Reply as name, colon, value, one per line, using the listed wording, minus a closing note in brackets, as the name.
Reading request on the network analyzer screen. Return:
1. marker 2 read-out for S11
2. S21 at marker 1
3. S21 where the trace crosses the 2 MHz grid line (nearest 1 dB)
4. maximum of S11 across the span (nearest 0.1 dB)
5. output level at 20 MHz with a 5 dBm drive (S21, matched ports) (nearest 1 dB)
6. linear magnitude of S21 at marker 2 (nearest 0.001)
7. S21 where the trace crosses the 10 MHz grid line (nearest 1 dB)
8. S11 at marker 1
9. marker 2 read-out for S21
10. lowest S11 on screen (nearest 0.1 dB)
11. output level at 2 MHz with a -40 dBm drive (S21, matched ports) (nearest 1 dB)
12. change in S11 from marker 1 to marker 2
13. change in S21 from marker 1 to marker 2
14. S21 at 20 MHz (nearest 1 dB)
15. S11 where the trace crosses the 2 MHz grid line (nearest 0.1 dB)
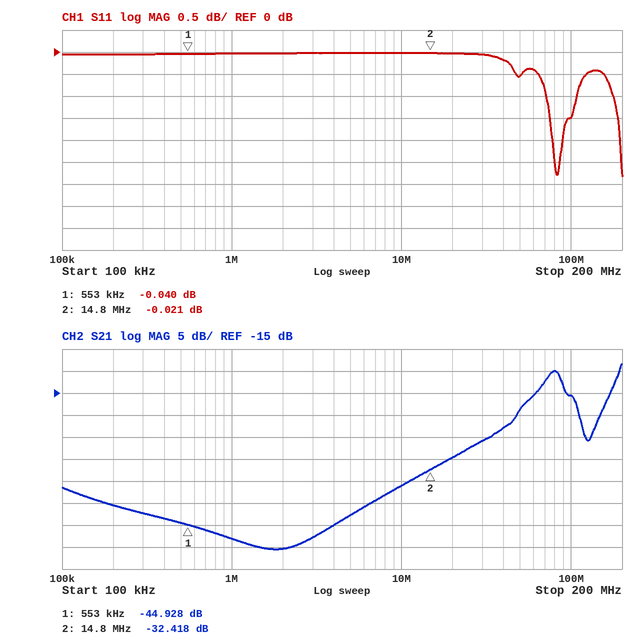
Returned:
marker 2 read-out for S11: -0.021 dB
S21 at marker 1: -44.928 dB
S21 where the trace crosses the 2 MHz grid line: -50 dB
maximum of S11 across the span: 0.0 dB
output level at 20 MHz with a 5 dBm drive (S21, matched ports): -25 dBm
linear magnitude of S21 at marker 2: 0.024
S21 where the trace crosses the 10 MHz grid line: -36 dB
S11 at marker 1: -0.040 dB
marker 2 read-out for S21: -32.418 dB
lowest S11 on screen: -2.8 dB
output level at 2 MHz with a -40 dBm drive (S21, matched ports): -90 dBm
change in S11 from marker 1 to marker 2: 0.019 dB
change in S21 from marker 1 to marker 2: 12.510 dB
S21 at 20 MHz: -30 dB
S11 where the trace crosses the 2 MHz grid line: 0.0 dB
